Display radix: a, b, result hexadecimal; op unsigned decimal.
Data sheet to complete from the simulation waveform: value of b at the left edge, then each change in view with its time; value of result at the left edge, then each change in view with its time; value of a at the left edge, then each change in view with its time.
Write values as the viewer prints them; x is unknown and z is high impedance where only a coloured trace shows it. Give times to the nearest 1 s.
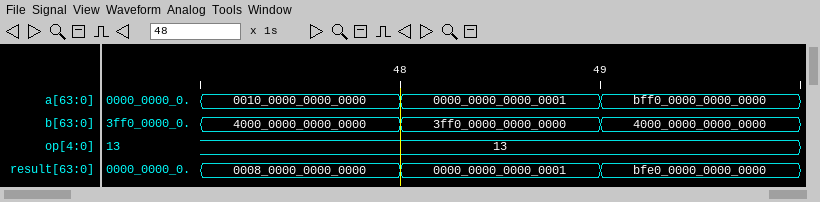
4000_0000_0000_0000, 3ff0_0000_0000_0000 at 48 s, 4000_0000_0000_0000 at 49 s
0008_0000_0000_0000, 0000_0000_0000_0001 at 48 s, bfe0_0000_0000_0000 at 49 s
0010_0000_0000_0000, 0000_0000_0000_0001 at 48 s, bff0_0000_0000_0000 at 49 s
